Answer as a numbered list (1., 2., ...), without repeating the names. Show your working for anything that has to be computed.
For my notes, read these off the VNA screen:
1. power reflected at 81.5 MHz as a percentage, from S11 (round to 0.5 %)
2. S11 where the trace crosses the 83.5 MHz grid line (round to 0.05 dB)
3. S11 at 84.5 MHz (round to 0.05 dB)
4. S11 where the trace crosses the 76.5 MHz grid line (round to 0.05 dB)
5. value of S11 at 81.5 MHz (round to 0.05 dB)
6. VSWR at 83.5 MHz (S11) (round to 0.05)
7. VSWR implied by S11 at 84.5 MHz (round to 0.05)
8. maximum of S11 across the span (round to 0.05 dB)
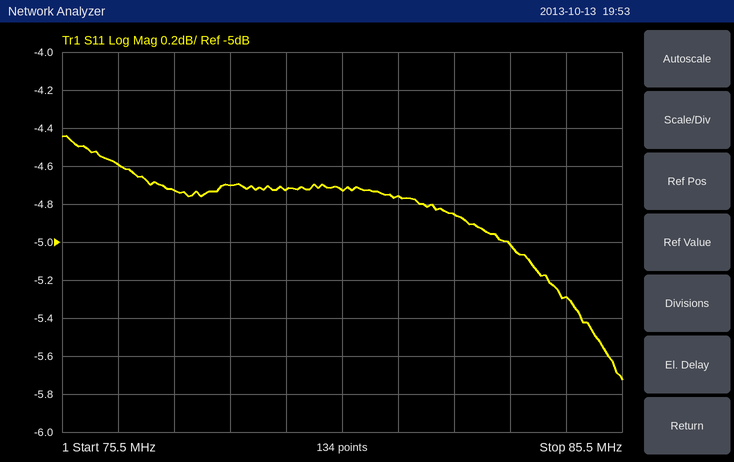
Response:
1. 10^(-4.75/10) ≈ 33.5 %
2. -5.00 dB
3. -5.30 dB
4. -4.60 dB
5. -4.75 dB
6. |Γ| = 10^(-5/20) = 0.5623; VSWR = (1 + 0.5623)/(1 − 0.5623) ≈ 3.57, so 3.55 to the nearest 0.05
7. |Γ| = 10^(-5.3/20) = 0.5433; VSWR = (1 + 0.5433)/(1 − 0.5433) ≈ 3.38, so 3.40 to the nearest 0.05
8. -4.45 dB
